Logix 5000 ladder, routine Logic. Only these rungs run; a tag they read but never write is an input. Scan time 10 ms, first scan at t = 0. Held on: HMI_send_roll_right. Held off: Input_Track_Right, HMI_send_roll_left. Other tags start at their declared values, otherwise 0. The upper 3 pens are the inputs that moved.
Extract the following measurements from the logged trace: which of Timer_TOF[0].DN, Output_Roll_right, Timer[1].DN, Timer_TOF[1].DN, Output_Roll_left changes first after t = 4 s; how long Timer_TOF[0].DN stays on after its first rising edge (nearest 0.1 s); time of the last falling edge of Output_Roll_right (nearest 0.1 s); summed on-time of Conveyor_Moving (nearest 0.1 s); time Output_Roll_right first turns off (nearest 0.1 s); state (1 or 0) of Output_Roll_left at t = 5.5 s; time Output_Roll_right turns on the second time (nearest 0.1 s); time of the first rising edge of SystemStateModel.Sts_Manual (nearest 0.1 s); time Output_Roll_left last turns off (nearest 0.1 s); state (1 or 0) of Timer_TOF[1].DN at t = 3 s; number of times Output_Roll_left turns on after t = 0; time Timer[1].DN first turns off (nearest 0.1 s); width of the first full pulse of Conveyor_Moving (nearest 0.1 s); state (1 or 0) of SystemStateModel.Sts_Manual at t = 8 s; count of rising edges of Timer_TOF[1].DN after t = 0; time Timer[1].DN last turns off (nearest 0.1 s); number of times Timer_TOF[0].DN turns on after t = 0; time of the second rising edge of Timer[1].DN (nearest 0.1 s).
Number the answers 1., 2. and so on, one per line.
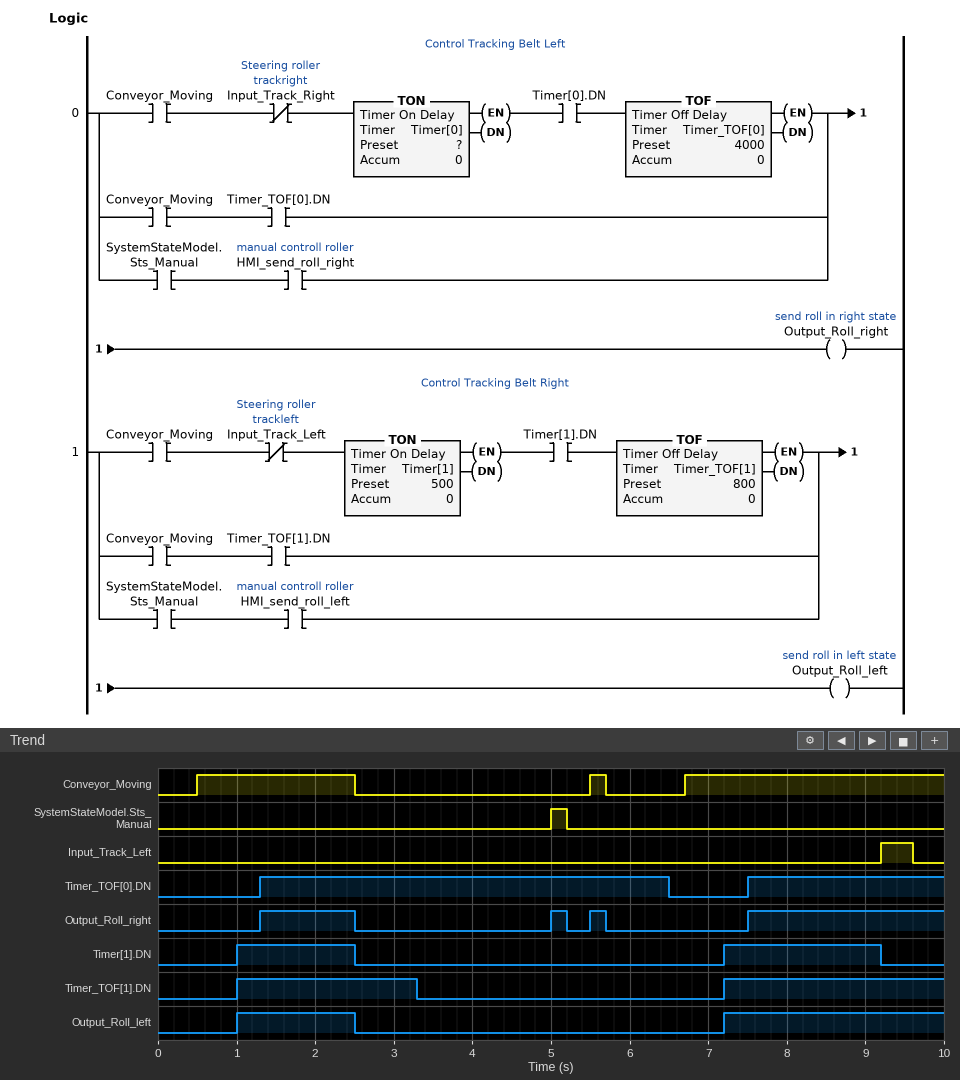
1. Output_Roll_right
2. 5.2 s
3. 5.7 s
4. 5.5 s
5. 2.5 s
6. 0
7. 5.0 s
8. 5.0 s
9. 2.5 s
10. 1
11. 2
12. 2.5 s
13. 2.0 s
14. 0
15. 2
16. 9.2 s
17. 2
18. 7.2 s
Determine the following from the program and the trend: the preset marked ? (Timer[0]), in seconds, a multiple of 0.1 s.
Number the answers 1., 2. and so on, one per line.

1. 0.8 s
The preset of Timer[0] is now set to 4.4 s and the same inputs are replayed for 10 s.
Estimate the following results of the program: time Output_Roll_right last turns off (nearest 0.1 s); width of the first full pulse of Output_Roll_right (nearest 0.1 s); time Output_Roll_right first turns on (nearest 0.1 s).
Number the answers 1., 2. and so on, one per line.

1. 5.2 s
2. 0.2 s
3. 5.0 s
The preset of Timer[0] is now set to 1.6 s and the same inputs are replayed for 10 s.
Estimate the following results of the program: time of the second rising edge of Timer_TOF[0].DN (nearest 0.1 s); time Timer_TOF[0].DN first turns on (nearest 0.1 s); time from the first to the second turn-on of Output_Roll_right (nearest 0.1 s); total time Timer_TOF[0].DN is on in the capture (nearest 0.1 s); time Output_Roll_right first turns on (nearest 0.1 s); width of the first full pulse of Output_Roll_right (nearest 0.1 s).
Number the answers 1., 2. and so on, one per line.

1. 8.3 s
2. 2.1 s
3. 2.9 s
4. 6.1 s
5. 2.1 s
6. 0.4 s
